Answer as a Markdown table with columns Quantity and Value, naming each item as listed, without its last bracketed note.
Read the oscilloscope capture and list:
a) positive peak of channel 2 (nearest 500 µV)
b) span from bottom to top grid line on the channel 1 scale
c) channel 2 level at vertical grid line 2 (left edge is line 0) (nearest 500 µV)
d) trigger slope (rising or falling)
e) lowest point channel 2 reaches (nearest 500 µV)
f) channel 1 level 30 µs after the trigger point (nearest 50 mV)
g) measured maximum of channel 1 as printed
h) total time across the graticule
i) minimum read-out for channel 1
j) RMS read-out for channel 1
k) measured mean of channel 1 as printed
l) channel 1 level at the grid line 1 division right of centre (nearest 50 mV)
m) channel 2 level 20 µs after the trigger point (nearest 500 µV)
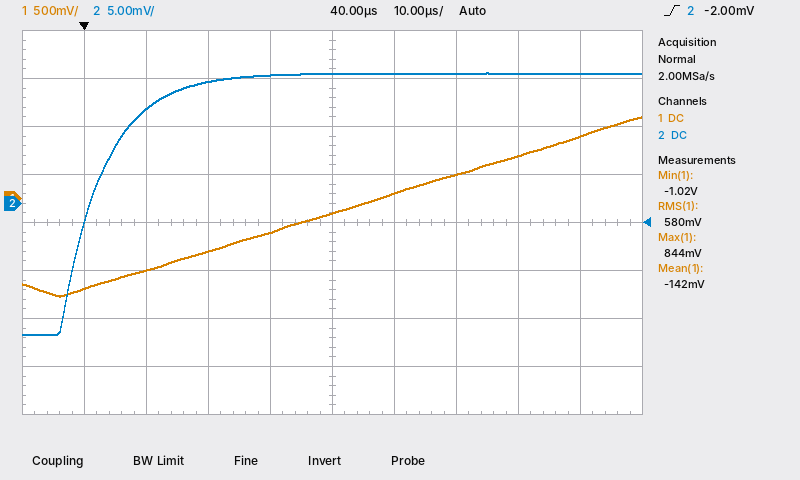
| Quantity | Value |
|---|---|
| positive peak of channel 2 | 13.5 mV |
| span from bottom to top grid line on the channel 1 scale | 4 V |
| channel 2 level at vertical grid line 2 (left edge is line 0) | 10.0 mV |
| trigger slope | rising |
| lowest point channel 2 reaches | -13.5 mV |
| channel 1 level 30 µs after the trigger point | -350 mV |
| measured maximum of channel 1 as printed | 844 mV |
| total time across the graticule | 100 µs |
| minimum read-out for channel 1 | -1.02 V |
| RMS read-out for channel 1 | 580 mV |
| measured mean of channel 1 as printed | -142 mV |
| channel 1 level at the grid line 1 division right of centre | 50 mV |
| channel 2 level 20 µs after the trigger point | 12.5 mV |
